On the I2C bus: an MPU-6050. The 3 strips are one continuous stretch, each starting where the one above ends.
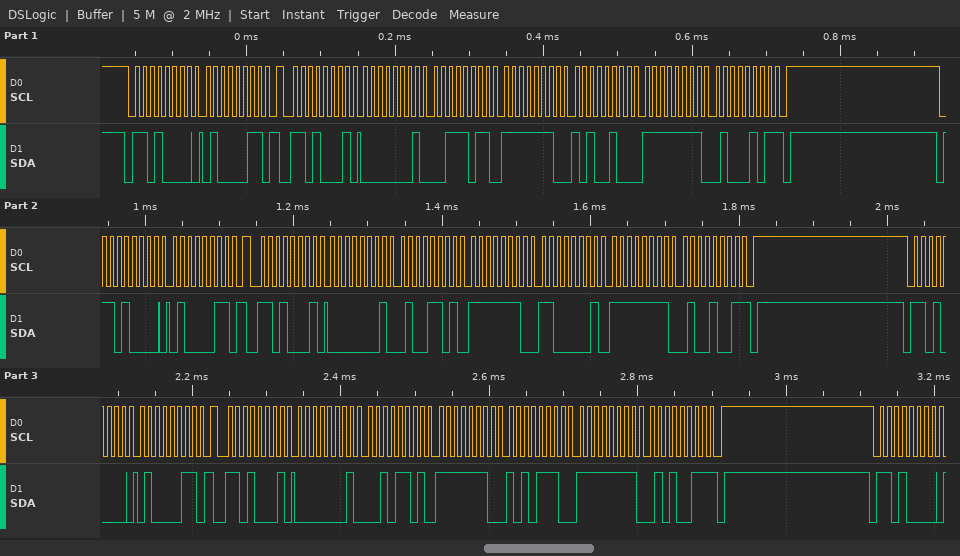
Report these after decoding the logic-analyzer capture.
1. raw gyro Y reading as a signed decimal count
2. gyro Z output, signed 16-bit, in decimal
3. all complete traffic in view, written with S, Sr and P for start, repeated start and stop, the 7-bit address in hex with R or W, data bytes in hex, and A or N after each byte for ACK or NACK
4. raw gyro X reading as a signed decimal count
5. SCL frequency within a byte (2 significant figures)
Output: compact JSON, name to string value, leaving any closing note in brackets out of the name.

{"raw gyro Y reading as a signed decimal count": "-348", "gyro Z output, signed 16-bit, in decimal": "-187", "all complete traffic in view, written with S, Sr and P for start, repeated start and stop, the 7-bit address in hex with R or W, data bytes in hex, and A or N after each byte for ACK or NACK": "S 68W A 43 A Sr 68R A 01 A 3B A FE A A4 A FF A 45 N P S 68W A 43 A Sr 68R A 01 A 4D A FE A C1 A FF A 49 N P S 68W A 43 A Sr 68R A 01 A 2D A FE A AE A FF A 53 N P S 68W A", "raw gyro X reading as a signed decimal count": "315", "SCL frequency within a byte": "100 kHz"}
